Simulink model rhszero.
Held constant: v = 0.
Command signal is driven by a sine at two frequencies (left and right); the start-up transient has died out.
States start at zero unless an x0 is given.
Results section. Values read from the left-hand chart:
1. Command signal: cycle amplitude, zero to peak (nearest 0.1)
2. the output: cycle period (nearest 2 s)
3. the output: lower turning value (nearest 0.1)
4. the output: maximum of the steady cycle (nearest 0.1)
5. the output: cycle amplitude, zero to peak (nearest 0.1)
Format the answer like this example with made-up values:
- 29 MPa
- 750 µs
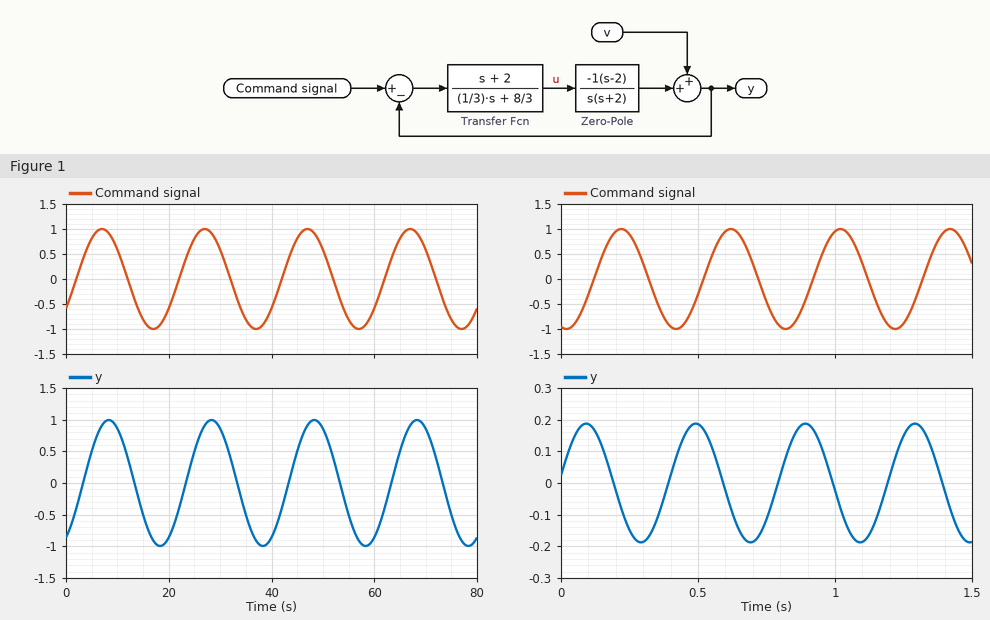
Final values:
- 1.0
- 20 s
- -1.0
- 1.0
- 1.0
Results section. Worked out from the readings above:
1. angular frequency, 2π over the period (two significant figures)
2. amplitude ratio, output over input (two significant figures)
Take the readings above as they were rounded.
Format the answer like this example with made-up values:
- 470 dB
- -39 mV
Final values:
- 0.31 rad/s
- 1.0
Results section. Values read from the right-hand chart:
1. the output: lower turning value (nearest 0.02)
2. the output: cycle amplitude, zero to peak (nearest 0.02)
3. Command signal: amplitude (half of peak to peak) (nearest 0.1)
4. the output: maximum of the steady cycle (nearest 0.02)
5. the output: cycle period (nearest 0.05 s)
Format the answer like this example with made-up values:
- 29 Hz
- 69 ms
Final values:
- -0.18
- 0.18
- 1.0
- 0.18
- 0.40 s
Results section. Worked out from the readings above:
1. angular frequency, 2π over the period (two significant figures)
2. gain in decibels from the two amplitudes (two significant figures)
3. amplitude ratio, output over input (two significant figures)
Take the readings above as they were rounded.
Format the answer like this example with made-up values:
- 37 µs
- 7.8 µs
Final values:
- 16 rad/s
- -15 dB
- 0.18
